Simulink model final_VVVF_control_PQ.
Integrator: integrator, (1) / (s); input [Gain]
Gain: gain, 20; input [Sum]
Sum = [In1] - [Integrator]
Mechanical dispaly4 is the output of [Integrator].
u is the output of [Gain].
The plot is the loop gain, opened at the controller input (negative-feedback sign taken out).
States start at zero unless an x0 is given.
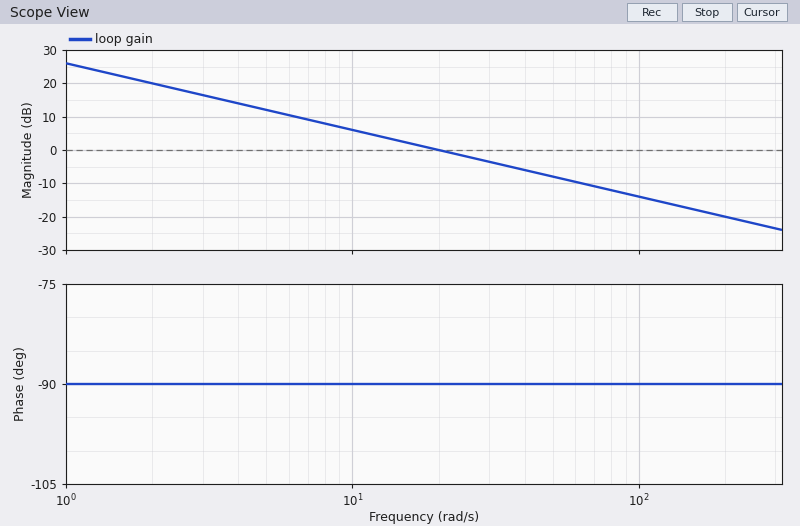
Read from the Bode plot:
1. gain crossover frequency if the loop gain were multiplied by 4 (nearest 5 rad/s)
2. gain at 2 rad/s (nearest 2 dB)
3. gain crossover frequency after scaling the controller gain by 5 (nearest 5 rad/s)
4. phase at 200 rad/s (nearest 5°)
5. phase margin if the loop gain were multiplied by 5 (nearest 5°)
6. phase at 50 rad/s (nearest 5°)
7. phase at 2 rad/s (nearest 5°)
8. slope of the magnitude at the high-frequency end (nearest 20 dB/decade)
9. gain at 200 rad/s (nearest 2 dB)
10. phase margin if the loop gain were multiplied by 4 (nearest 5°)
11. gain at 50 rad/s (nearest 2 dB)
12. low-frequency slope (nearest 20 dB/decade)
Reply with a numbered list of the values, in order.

1. 80 rad/s
2. 20 dB
3. 100 rad/s
4. -90°
5. 90°
6. -90°
7. -90°
8. -20 dB/decade
9. -20 dB
10. 90°
11. -8 dB
12. -20 dB/decade
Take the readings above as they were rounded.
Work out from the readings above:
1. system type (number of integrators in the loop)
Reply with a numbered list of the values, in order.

1. 1
